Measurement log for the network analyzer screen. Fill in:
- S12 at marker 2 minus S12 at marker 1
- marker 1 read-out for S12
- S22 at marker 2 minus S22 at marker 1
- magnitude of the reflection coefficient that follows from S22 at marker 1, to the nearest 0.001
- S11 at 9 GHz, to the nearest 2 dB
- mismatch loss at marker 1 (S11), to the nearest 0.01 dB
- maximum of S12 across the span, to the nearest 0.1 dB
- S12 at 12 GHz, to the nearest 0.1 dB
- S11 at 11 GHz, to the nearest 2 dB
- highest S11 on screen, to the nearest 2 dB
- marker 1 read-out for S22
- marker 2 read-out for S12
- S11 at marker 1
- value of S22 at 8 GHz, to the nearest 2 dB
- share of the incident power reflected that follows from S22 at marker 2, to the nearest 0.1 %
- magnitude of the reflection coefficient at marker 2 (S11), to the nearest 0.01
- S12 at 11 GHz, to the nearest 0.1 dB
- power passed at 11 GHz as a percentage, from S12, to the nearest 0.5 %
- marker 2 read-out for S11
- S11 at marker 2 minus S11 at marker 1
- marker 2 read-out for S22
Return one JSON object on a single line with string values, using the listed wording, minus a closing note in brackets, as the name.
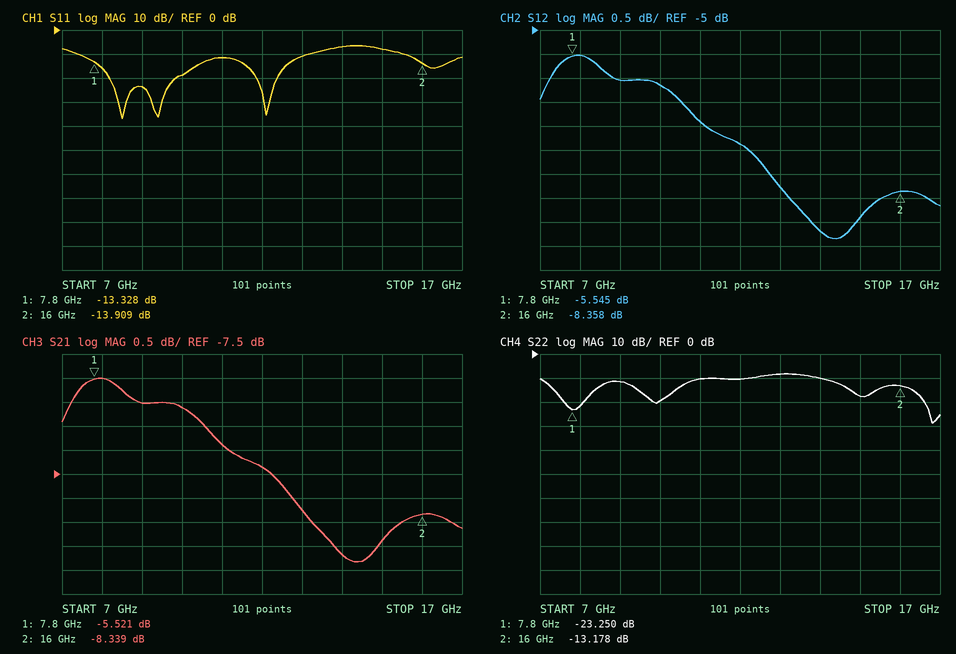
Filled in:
{"S12 at marker 2 minus S12 at marker 1": "-2.813 dB", "marker 1 read-out for S12": "-5.545 dB", "S22 at marker 2 minus S22 at marker 1": "10.072 dB", "magnitude of the reflection coefficient that follows from S22 at marker 1, to the nearest 0.001": "0.069", "S11 at 9 GHz, to the nearest 2 dB": "-24 dB", "mismatch loss at marker 1 (S11), to the nearest 0.01 dB": "0.21 dB", "maximum of S12 across the span, to the nearest 0.1 dB": "-5.5 dB", "S12 at 12 GHz, to the nearest 0.1 dB": "-7.4 dB", "S11 at 11 GHz, to the nearest 2 dB": "-12 dB", "highest S11 on screen, to the nearest 2 dB": "-6 dB", "marker 1 read-out for S22": "-23.250 dB", "marker 2 read-out for S12": "-8.358 dB", "S11 at marker 1": "-13.328 dB", "value of S22 at 8 GHz, to the nearest 2 dB": "-22 dB", "share of the incident power reflected that follows from S22 at marker 2, to the nearest 0.1 %": "4.8 %", "magnitude of the reflection coefficient at marker 2 (S11), to the nearest 0.01": "0.20", "S12 at 11 GHz, to the nearest 0.1 dB": "-6.9 dB", "power passed at 11 GHz as a percentage, from S12, to the nearest 0.5 %": "20.5 %", "marker 2 read-out for S11": "-13.909 dB", "S11 at marker 2 minus S11 at marker 1": "-0.581 dB", "marker 2 read-out for S22": "-13.178 dB"}
